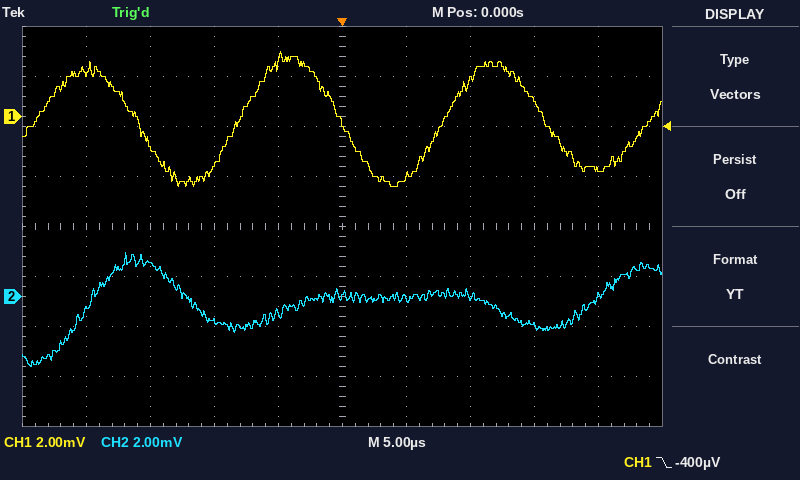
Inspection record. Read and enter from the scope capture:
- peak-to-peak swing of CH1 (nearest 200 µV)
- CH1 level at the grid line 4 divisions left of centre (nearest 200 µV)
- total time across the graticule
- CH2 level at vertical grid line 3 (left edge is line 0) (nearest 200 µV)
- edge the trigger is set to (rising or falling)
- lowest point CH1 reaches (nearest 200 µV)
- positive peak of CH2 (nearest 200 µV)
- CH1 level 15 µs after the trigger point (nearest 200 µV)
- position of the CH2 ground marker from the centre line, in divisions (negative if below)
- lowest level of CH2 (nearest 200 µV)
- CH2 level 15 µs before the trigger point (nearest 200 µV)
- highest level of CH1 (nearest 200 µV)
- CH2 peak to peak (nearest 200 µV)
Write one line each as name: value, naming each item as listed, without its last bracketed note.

peak-to-peak swing of CH1: 5.4 mV
CH1 level at the grid line 4 divisions left of centre: 1.8 mV
total time across the graticule: 50 µs
CH2 level at vertical grid line 3 (left edge is line 0): -1.0 mV
edge the trigger is set to: falling
lowest point CH1 reaches: -2.8 mV
positive peak of CH2: 1.8 mV
CH1 level 15 µs after the trigger point: 600 µV
position of the CH2 ground marker from the centre line, in divisions: -1.4 div
lowest level of CH2: -2.8 mV
CH2 level 15 µs before the trigger point: 1.4 mV
highest level of CH1: 2.6 mV
CH2 peak to peak: 4.6 mV
